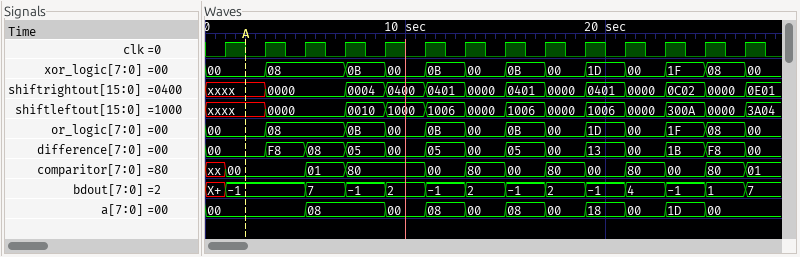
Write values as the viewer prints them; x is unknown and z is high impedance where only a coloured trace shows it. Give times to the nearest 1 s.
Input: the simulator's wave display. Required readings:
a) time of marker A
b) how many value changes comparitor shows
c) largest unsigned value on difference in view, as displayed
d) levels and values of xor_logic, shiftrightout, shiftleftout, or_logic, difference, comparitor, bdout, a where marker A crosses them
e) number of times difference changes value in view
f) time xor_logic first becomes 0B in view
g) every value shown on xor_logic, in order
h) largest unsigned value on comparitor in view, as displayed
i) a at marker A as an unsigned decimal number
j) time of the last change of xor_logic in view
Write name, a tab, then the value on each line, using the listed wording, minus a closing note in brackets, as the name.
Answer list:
time of marker A	2 s
how many value changes comparitor shows	12
largest unsigned value on difference in view, as displayed	F8
levels and values of xor_logic, shiftrightout, shiftleftout, or_logic, difference, comparitor, bdout, a where marker A crosses them	xor_logic=00, shiftrightout=xxxx, shiftleftout=xxxx, or_logic=00, difference=00, comparitor=00, bdout=-1, a=00
number of times difference changes value in view	13
time xor_logic first becomes 0B in view	7 s
every value shown on xor_logic, in order	00, 08, 0B, 00, 0B, 00, 0B, 00, 1D, 00, 1F, 08, 00
largest unsigned value on comparitor in view, as displayed	80
a at marker A as an unsigned decimal number	0
time of the last change of xor_logic in view	27 s
